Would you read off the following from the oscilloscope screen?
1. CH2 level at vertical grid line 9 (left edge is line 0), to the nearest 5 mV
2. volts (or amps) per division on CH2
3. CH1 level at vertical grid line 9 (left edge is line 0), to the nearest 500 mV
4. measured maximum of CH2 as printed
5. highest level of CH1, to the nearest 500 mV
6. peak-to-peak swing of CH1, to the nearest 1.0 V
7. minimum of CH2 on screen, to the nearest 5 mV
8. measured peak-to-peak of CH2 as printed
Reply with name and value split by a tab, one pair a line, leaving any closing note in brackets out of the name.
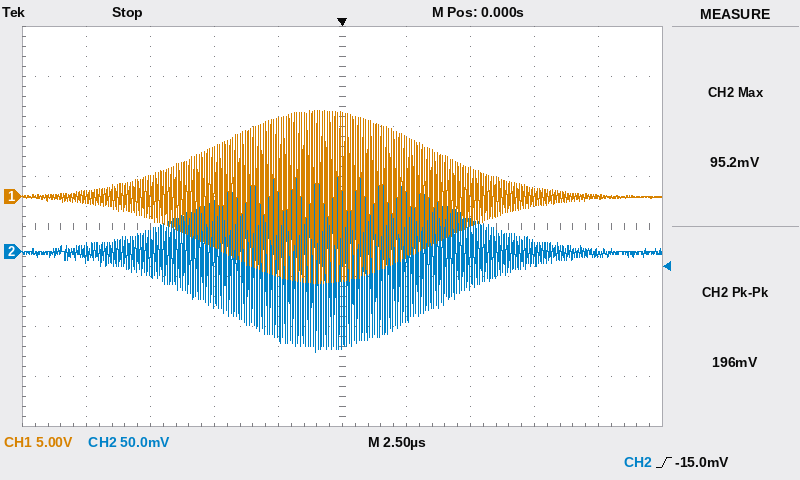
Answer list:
CH2 level at vertical grid line 9 (left edge is line 0), to the nearest 5 mV	0 mV
volts (or amps) per division on CH2	50 mV
CH1 level at vertical grid line 9 (left edge is line 0), to the nearest 500 mV	0.0 V
measured maximum of CH2 as printed	95.2 mV
highest level of CH1, to the nearest 500 mV	8.5 V
peak-to-peak swing of CH1, to the nearest 1.0 V	17.0 V
minimum of CH2 on screen, to the nearest 5 mV	-100 mV
measured peak-to-peak of CH2 as printed	196 mV
